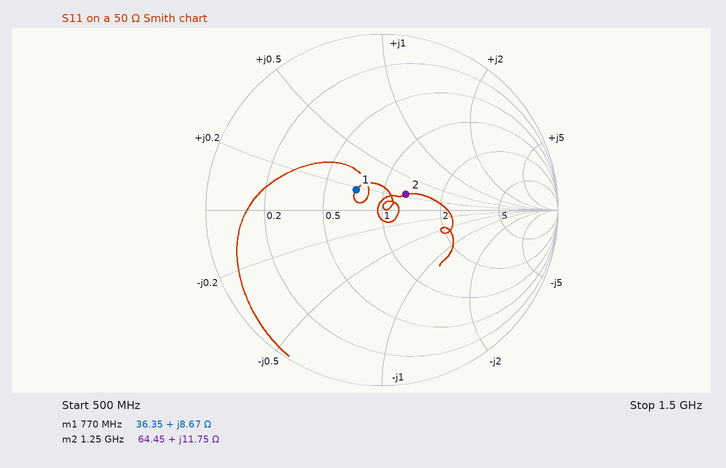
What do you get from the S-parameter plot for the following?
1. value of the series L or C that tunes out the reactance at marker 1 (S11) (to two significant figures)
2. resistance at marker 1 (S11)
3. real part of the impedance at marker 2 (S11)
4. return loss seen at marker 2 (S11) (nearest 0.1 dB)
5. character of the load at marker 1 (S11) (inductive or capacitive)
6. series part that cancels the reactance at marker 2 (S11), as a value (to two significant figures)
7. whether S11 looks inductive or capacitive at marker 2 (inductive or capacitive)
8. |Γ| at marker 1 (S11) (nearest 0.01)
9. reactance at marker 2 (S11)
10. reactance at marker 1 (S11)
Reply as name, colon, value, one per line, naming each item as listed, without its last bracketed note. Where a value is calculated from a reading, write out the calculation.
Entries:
value of the series L or C that tunes out the reactance at marker 1 (S11): C = 1/(2π × 770 MHz × 8.67 Ω) ≈ 24 pF
resistance at marker 1: 36.35 Ω
real part of the impedance at marker 2: 64.45 Ω
return loss seen at marker 2 (S11): 15.8 dB
character of the load at marker 1 (S11): inductive
series part that cancels the reactance at marker 2 (S11), as a value: C = 1/(2π × 1.25 GHz × 11.75 Ω) ≈ 11 pF
whether S11 looks inductive or capacitive at marker 2: inductive
|Γ| at marker 1 (S11): 0.19
reactance at marker 2: +11.75 Ω
reactance at marker 1: +8.67 Ω
